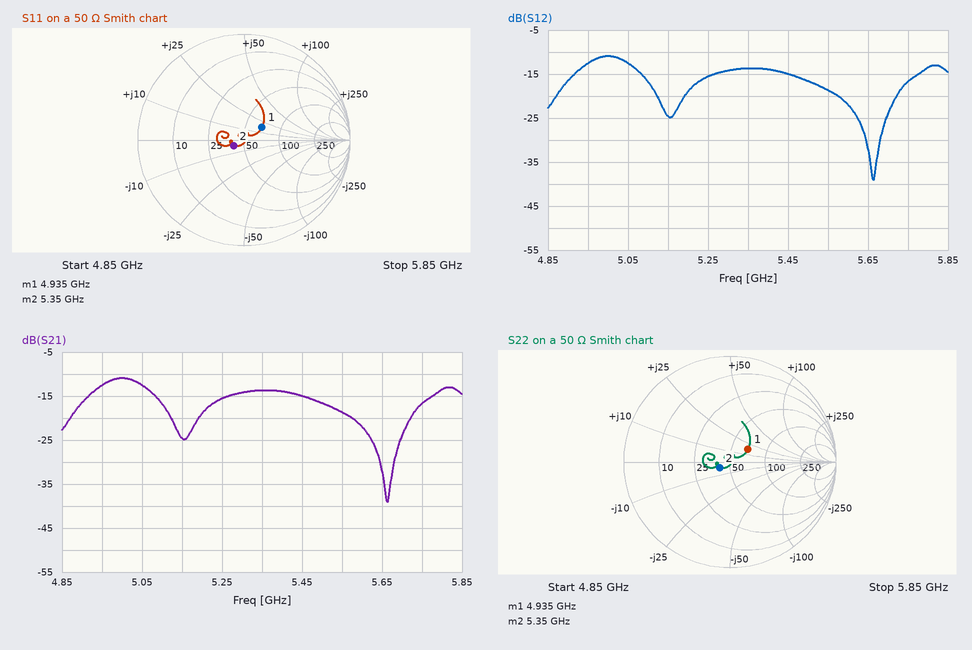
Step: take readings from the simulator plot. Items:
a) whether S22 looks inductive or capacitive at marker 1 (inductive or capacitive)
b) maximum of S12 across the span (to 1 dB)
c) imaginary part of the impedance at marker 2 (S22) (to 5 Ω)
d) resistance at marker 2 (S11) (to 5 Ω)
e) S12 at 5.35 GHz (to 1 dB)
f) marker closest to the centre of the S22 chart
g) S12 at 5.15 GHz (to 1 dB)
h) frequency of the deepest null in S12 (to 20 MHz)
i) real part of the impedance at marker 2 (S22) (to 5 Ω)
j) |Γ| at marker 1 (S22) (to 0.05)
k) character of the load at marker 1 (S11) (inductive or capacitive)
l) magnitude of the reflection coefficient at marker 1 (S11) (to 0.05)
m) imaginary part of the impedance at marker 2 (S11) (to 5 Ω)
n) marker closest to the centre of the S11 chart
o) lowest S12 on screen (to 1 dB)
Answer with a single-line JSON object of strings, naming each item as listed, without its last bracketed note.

{"whether S22 looks inductive or capacitive at marker 1": "inductive", "maximum of S12 across the span": "-11 dB", "imaginary part of the impedance at marker 2 (S22)": "-5 Ω", "resistance at marker 2 (S11)": "40 Ω", "S12 at 5.35 GHz": "-14 dB", "marker closest to the centre of the S22 chart": "marker 2", "S12 at 5.15 GHz": "-25 dB", "frequency of the deepest null in S12": "5.66 GHz", "real part of the impedance at marker 2 (S22)": "40 Ω", "|Γ| at marker 1 (S22)": "0.20", "character of the load at marker 1 (S11)": "inductive", "magnitude of the reflection coefficient at marker 1 (S11)": "0.20", "imaginary part of the impedance at marker 2 (S11)": "-5 Ω", "marker closest to the centre of the S11 chart": "marker 2", "lowest S12 on screen": "-39 dB"}
